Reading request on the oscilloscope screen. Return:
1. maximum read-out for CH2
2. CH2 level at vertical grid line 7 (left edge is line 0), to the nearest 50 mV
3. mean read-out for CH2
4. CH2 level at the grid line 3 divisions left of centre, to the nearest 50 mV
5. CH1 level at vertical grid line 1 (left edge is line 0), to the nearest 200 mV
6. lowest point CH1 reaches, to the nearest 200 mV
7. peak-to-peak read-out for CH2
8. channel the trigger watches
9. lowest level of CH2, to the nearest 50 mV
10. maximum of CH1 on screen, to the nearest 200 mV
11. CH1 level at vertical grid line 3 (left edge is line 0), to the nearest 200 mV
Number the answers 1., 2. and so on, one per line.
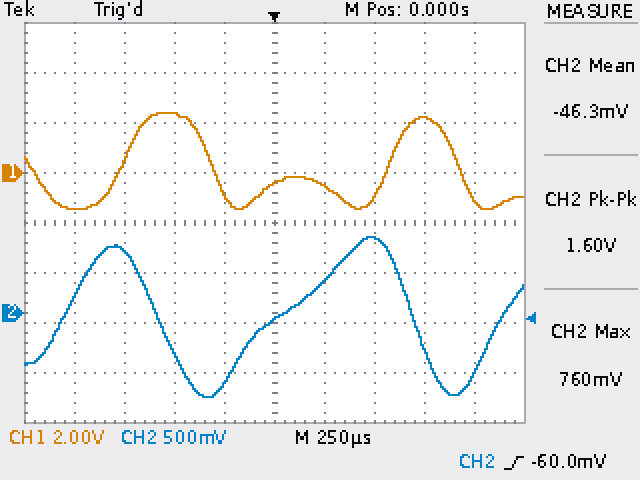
1. 760 mV
2. 750 mV
3. -46.3 mV
4. 600 mV
5. -1.4 V
6. -1.4 V
7. 1.60 V
8. CH2
9. -850 mV
10. 2.4 V
11. 2.4 V
